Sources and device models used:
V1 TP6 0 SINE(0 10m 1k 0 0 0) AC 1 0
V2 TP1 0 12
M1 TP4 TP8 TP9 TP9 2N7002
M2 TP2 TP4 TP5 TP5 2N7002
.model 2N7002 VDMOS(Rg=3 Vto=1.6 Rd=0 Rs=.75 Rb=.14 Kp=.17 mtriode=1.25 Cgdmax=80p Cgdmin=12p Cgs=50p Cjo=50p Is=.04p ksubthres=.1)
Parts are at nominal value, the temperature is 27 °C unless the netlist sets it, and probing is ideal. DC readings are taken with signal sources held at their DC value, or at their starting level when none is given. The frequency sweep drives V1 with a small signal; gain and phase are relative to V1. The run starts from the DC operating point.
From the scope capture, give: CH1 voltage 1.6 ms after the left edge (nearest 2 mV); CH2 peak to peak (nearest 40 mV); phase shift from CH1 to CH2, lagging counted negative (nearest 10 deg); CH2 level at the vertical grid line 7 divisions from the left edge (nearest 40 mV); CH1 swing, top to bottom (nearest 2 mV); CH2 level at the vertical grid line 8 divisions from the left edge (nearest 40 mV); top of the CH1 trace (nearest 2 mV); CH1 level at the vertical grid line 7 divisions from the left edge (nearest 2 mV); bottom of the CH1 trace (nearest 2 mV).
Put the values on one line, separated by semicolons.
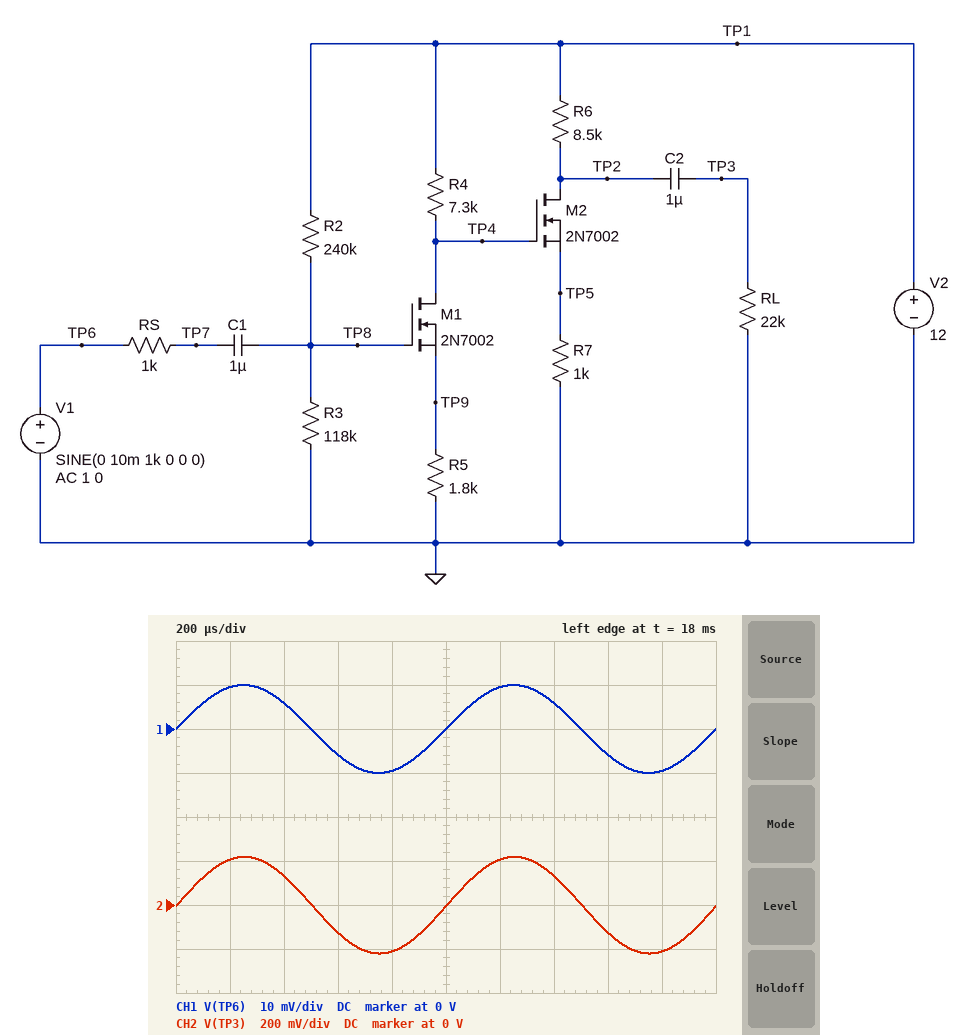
-6 mV; 440 mV; 0 deg; 120 mV; 20 mV; -120 mV; 10 mV; 6 mV; -10 mV
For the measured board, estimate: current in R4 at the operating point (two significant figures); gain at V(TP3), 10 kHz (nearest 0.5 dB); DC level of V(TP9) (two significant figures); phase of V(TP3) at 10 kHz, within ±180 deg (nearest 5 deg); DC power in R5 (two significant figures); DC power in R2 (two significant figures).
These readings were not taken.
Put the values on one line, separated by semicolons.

1.3 mA; 26.5 dB; 2.3 V; -15 deg; 2.9 mW; 270 µW
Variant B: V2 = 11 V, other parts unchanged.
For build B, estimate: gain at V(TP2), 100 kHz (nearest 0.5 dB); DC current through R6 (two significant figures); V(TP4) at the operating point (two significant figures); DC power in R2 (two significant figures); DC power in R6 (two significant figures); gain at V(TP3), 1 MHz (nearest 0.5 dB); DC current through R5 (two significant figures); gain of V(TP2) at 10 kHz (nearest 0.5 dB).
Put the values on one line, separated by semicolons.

-13.5 dB; 1.2 mA; 3.1 V; 230 µW; 11 mW; -11.0 dB; 1.1 mA; -15.5 dB
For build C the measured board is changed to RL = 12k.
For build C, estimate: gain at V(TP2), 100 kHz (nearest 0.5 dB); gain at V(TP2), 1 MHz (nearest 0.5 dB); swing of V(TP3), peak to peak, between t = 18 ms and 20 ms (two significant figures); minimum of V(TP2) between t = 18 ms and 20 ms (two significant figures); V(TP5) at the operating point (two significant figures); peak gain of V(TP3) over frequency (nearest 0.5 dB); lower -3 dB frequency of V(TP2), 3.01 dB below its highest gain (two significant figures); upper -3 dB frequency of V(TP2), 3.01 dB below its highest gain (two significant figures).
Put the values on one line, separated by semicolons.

17.0 dB; -1.0 dB; 360 mV; 2.3 V; 1.1 V; 25.0 dB; 1.5 Hz; 74 Hz
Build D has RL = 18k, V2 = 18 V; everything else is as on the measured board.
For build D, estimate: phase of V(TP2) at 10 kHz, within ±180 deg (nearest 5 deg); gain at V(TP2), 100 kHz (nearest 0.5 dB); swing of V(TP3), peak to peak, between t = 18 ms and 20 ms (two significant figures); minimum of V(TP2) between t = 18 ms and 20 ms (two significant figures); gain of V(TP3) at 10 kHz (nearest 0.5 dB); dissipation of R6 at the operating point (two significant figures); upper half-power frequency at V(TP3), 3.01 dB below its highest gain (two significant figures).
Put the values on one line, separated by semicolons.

-50 deg; -6.0 dB; 1.4 mV; 2.3 V; -20.5 dB; 29 mW; 1.6 MHz
